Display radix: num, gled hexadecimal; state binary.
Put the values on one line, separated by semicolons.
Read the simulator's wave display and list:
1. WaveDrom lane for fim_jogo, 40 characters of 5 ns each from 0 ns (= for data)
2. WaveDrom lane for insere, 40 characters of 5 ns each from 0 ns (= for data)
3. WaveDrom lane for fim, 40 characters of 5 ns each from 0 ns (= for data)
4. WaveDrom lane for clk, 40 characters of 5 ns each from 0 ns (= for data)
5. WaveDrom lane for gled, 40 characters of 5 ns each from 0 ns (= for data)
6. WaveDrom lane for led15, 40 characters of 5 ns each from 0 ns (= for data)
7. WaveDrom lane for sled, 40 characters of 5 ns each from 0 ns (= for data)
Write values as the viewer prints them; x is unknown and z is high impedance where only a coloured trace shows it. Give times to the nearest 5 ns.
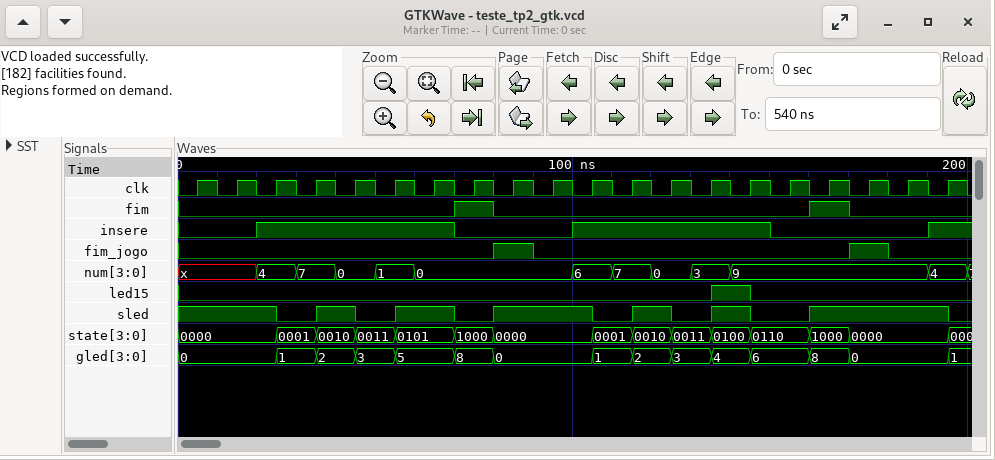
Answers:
{name: 'fim_jogo', wave: '0...............1.0...............1.0...'}; {name: 'insere', wave: '0...1.........0.....1.........0.......1.'}; {name: 'fim', wave: '0.............1.0...............1.0.....'}; {name: 'clk', wave: '0101010101010101010101010101010101010101'}; {name: 'gled', wave: '=....=.=.=.=..=.=....=.=.=.=.=..=.=....=', data: '0 1 2 3 5 8 0 1 2 3 4 6 8 0 1'}; {name: 'led15', wave: '0..........................1.0..........'}; {name: 'sled', wave: '1....0.1.0.1..0.1....0.1.0.1.0..1......0'}
